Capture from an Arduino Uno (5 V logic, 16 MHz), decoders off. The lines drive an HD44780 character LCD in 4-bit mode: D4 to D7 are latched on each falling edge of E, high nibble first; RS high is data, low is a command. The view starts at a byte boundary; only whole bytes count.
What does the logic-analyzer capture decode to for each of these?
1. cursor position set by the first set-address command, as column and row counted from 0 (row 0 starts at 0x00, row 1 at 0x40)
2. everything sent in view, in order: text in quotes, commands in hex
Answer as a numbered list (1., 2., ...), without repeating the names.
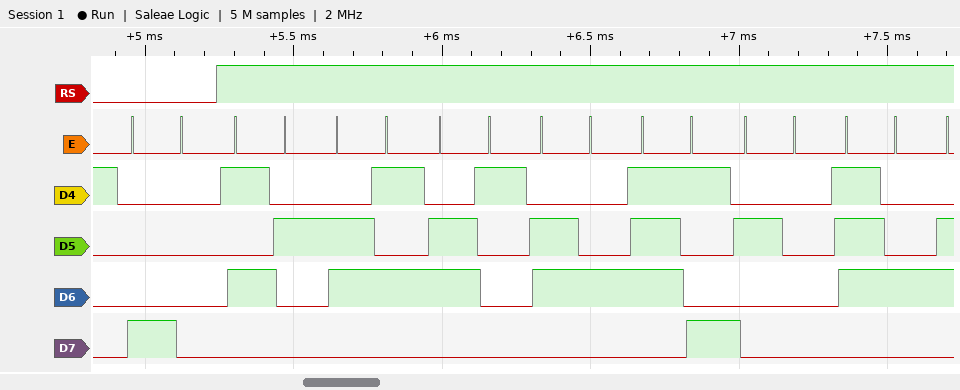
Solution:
1. column 0, row 0
2. 0x80 "Ready t"
